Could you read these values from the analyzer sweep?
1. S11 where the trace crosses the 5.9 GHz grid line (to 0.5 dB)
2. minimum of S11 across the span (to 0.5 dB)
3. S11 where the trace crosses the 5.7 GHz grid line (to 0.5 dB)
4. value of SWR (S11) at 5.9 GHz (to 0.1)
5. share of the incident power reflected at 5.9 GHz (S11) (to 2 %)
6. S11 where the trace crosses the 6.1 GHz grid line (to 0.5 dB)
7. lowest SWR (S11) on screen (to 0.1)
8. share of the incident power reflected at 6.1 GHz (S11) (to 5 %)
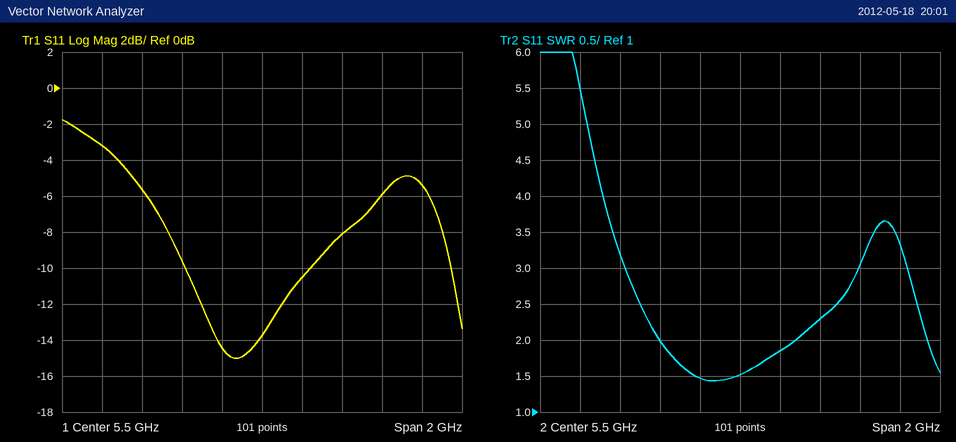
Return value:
-8.0 dB
-15.0 dB
-10.5 dB
2.3
16 %
-6.0 dB
1.4
25 %
